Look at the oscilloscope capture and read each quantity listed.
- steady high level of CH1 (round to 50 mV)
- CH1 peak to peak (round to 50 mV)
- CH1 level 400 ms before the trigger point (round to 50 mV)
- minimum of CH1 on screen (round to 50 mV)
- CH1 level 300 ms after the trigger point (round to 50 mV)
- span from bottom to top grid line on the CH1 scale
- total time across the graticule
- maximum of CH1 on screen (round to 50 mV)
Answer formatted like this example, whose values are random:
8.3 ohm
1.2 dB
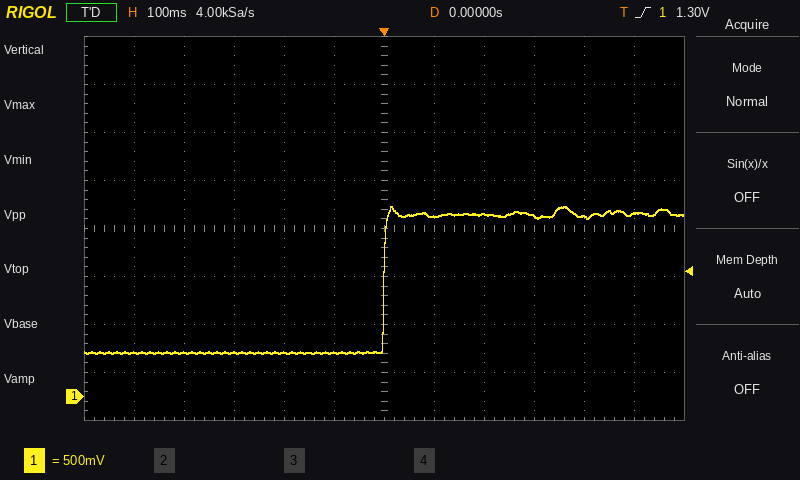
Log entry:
1.90 V
1.55 V
450 mV
450 mV
1.90 V
4 V
1.2 s
2.00 V
